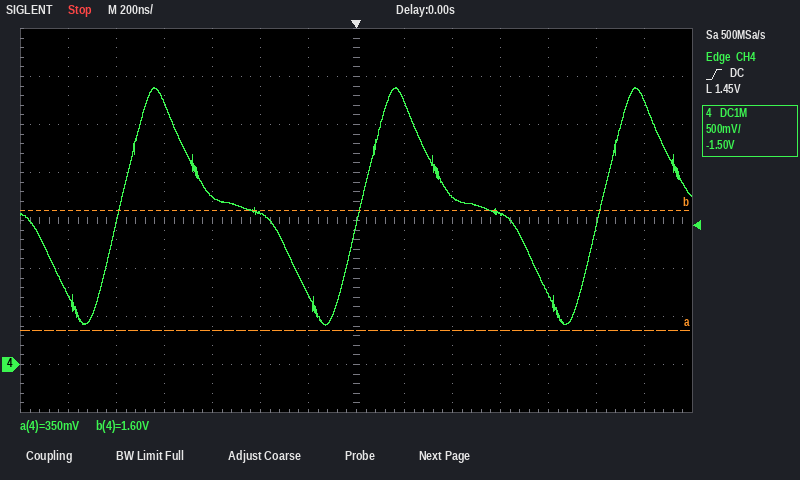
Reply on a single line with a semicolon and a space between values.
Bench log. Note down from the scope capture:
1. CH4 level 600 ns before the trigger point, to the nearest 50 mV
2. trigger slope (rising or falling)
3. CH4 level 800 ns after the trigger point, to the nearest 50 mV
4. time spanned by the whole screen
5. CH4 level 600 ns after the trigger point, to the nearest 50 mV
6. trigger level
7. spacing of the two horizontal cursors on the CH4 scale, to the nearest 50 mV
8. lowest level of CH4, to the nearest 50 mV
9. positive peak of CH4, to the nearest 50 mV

1.75 V; rising; 750 mV; 2.8 µs; 1.55 V; 1.45 V; 1.25 V; 400 mV; 2.90 V
